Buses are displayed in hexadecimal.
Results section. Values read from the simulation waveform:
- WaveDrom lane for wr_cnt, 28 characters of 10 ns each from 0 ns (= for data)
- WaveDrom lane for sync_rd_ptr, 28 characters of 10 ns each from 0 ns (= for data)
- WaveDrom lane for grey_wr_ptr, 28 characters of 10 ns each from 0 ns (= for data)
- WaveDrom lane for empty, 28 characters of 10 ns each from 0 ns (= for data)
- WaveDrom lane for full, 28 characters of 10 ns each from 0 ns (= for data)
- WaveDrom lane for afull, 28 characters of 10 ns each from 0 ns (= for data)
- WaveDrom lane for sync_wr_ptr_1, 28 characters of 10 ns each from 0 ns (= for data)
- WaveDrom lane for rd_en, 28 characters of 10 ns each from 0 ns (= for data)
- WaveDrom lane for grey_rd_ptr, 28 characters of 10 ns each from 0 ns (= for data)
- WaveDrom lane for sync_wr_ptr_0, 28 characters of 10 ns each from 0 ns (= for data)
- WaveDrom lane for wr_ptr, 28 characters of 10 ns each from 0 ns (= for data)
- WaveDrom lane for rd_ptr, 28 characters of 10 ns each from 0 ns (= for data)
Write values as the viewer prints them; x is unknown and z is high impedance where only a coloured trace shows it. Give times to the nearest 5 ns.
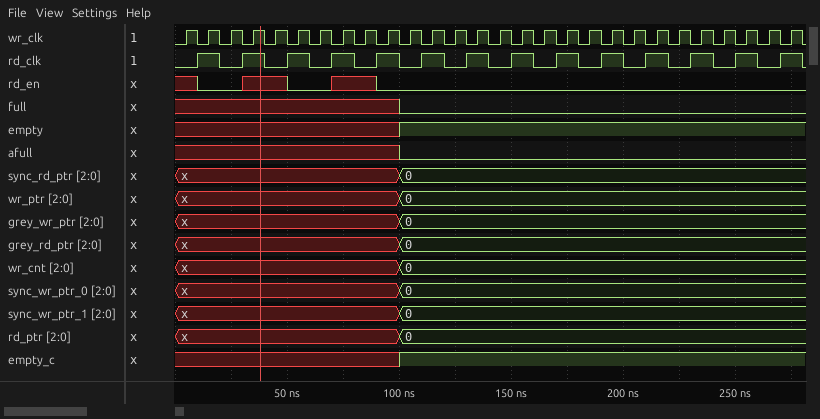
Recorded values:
{name: 'wr_cnt', wave: 'x.........=.................', data: '0'}
{name: 'sync_rd_ptr', wave: 'x.........=.................', data: '0'}
{name: 'grey_wr_ptr', wave: 'x.........=.................', data: '0'}
{name: 'empty', wave: 'x.........1.................'}
{name: 'full', wave: 'x.........0.................'}
{name: 'afull', wave: 'x.........0.................'}
{name: 'sync_wr_ptr_1', wave: 'x.........=.................', data: '0'}
{name: 'rd_en', wave: 'x0.x.0.x.0..................'}
{name: 'grey_rd_ptr', wave: 'x.........=.................', data: '0'}
{name: 'sync_wr_ptr_0', wave: 'x.........=.................', data: '0'}
{name: 'wr_ptr', wave: 'x.........=.................', data: '0'}
{name: 'rd_ptr', wave: 'x.........=.................', data: '0'}
